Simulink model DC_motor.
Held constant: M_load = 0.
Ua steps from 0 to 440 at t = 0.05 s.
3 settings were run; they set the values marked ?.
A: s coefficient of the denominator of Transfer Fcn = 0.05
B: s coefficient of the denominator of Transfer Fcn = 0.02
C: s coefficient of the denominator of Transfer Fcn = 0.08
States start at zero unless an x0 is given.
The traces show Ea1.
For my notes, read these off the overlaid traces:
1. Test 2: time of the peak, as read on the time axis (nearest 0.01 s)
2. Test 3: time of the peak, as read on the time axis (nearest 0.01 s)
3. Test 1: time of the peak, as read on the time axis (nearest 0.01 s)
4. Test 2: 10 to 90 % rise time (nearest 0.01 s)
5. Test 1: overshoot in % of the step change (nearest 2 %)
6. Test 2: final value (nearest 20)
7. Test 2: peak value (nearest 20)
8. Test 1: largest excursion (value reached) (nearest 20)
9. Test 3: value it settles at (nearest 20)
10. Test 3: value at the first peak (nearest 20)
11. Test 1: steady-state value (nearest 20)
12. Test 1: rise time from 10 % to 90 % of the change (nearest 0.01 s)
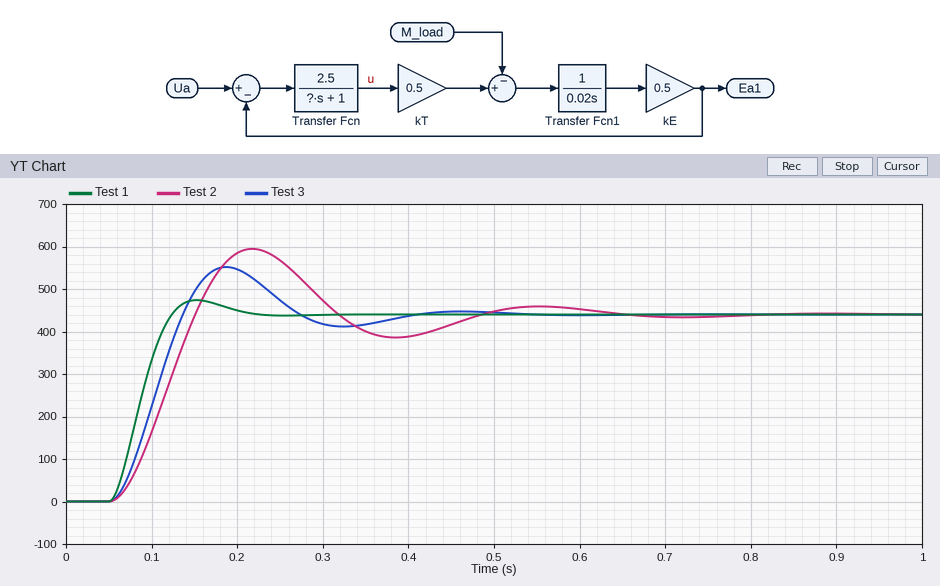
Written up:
0.22 s
0.19 s
0.15 s
0.07 s
8 %
440
600
480
440
560
440
0.05 s
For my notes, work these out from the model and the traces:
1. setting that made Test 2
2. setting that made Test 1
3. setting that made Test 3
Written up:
C
B
A
